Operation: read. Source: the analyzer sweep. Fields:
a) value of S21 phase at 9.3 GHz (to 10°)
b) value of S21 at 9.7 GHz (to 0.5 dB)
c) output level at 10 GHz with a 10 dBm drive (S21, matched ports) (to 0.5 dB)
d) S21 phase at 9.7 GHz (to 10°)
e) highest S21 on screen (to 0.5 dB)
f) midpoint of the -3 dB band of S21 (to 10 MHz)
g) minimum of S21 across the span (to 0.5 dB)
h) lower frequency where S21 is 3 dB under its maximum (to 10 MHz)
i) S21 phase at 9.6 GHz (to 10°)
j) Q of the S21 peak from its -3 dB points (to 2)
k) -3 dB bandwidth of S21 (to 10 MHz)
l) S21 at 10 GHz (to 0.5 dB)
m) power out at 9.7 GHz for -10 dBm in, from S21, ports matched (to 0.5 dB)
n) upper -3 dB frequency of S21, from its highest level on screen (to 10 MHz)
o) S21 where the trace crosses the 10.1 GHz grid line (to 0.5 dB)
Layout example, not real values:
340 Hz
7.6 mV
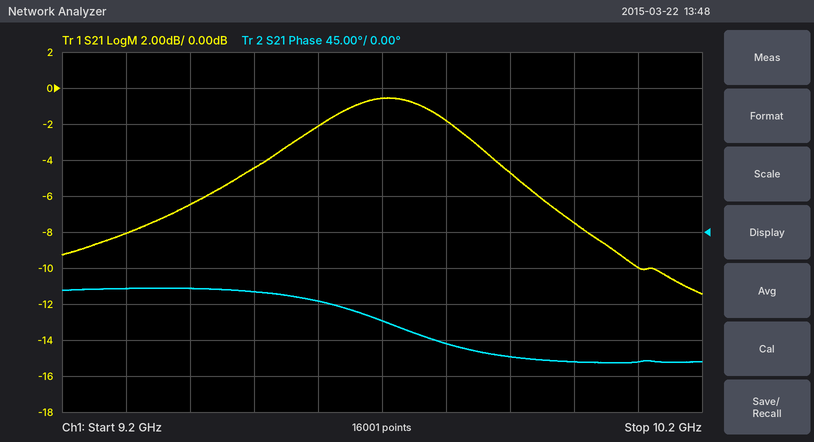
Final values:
-70°
-0.5 dB
2.5 dBm
-110°
-0.5 dB
9.70 GHz
-11.5 dB
9.54 GHz
-90°
30
320 MHz
-7.5 dB
-10.5 dBm
9.86 GHz
-10.0 dB
